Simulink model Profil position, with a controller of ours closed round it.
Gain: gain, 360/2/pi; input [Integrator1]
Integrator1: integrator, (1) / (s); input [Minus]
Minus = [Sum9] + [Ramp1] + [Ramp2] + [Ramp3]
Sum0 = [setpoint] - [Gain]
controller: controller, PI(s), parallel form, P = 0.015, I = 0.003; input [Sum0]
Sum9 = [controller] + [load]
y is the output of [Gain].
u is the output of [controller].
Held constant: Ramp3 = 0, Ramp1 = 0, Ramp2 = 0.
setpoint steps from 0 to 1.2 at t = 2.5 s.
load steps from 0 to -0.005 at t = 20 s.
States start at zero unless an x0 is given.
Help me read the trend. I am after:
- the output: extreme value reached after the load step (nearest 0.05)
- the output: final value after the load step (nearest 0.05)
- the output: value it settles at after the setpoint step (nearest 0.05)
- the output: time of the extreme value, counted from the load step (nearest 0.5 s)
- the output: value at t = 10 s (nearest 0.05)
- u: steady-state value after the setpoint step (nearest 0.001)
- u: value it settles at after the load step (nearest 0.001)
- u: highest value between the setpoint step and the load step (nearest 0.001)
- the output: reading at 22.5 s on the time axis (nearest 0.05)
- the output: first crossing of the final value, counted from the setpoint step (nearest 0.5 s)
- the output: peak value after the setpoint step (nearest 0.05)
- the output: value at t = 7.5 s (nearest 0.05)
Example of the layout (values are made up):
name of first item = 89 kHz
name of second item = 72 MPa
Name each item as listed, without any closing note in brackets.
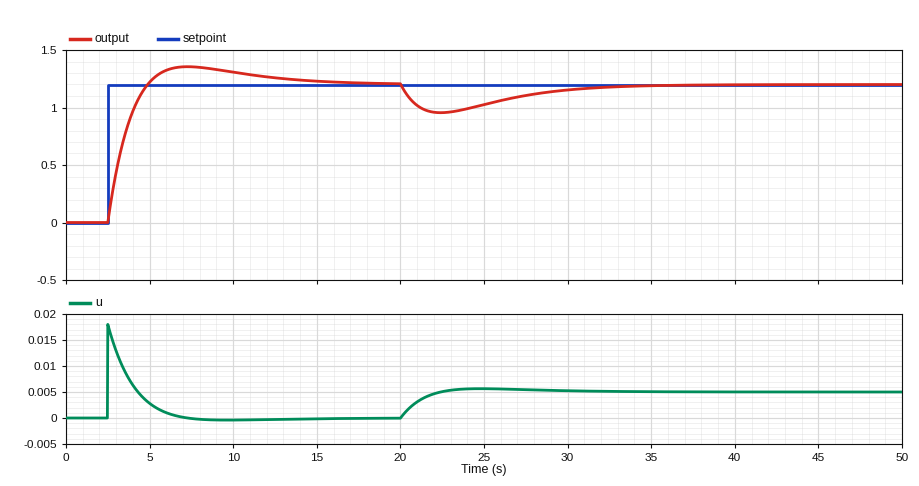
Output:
the output: extreme value reached after the load step = 0.95
the output: final value after the load step = 1.20
the output: value it settles at after the setpoint step = 1.20
the output: time of the extreme value, counted from the load step = 2.5 s
the output: value at t = 10 s = 1.30
u: steady-state value after the setpoint step = 0.000
u: value it settles at after the load step = 0.005
u: highest value between the setpoint step and the load step = 0.018
the output: reading at 22.5 s on the time axis = 0.95
the output: first crossing of the final value, counted from the setpoint step = 2.5 s
the output: peak value after the setpoint step = 1.35
the output: value at t = 7.5 s = 1.35
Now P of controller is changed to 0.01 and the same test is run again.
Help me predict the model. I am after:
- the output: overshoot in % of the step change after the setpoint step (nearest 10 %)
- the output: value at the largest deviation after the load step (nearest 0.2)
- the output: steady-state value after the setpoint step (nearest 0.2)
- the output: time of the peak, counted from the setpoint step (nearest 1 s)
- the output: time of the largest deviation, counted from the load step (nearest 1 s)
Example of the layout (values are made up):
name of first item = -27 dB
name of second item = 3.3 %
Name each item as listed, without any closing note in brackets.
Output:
the output: overshoot in % of the step change after the setpoint step = 20 %
the output: value at the largest deviation after the load step = 0.8
the output: steady-state value after the setpoint step = 1.2
the output: time of the peak, counted from the setpoint step = 5 s
the output: time of the largest deviation, counted from the load step = 3 s
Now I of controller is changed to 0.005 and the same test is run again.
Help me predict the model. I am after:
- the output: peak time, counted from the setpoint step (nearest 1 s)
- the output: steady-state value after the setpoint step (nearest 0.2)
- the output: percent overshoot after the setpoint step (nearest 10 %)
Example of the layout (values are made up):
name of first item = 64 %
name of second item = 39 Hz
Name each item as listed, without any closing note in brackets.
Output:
the output: peak time, counted from the setpoint step = 4 s
the output: steady-state value after the setpoint step = 1.2
the output: percent overshoot after the setpoint step = 20 %
